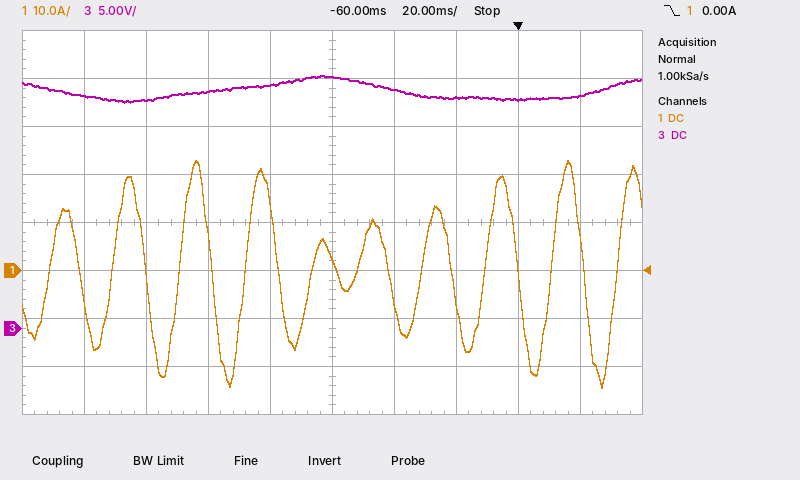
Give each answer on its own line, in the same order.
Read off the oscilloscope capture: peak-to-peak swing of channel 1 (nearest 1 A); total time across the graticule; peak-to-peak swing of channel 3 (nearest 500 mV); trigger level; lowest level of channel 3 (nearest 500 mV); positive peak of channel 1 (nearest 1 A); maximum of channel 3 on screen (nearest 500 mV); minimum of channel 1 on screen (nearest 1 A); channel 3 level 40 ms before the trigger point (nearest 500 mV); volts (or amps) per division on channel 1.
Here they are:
47 A
200 ms
3.0 V
0.00 A
23.5 V
23 A
26.5 V
-24 A
25.0 V
10 A
